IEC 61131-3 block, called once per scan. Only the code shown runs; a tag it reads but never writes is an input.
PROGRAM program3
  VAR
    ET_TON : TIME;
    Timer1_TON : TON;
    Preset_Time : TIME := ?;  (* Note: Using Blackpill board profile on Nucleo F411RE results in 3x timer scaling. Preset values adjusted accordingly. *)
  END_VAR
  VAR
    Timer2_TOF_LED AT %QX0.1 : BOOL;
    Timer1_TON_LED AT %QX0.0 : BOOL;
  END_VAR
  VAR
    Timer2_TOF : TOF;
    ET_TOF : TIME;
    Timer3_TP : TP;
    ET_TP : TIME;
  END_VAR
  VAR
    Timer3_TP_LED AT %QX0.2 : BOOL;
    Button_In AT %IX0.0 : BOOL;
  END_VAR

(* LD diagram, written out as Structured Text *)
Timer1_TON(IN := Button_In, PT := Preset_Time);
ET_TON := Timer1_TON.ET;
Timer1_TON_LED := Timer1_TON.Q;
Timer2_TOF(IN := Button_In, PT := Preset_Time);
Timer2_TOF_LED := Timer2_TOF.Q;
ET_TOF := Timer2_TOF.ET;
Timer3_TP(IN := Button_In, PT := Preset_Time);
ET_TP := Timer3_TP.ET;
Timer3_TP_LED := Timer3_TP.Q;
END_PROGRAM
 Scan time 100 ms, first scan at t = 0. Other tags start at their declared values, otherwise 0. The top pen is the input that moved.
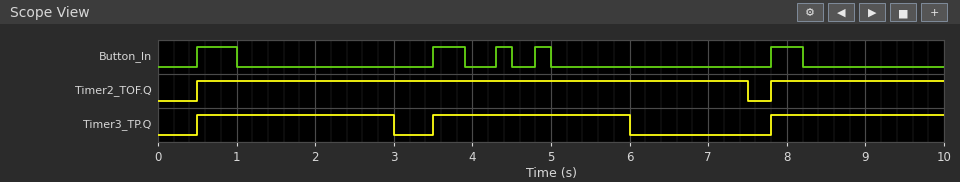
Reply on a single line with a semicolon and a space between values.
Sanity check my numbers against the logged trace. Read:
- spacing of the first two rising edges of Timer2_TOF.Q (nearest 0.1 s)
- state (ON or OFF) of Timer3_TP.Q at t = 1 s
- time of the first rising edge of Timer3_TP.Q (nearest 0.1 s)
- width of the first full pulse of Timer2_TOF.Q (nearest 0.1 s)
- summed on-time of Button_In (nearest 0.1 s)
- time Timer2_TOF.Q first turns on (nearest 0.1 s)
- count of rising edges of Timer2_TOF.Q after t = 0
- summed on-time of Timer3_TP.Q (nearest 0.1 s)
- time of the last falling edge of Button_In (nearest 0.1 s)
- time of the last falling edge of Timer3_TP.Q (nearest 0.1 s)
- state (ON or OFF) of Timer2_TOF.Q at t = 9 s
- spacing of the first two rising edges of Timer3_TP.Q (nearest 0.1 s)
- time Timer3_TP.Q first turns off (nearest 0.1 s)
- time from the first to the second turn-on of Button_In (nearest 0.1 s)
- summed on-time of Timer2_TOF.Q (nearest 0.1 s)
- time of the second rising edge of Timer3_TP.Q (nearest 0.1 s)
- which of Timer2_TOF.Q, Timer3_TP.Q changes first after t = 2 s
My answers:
7.3 s; ON; 0.5 s; 7.0 s; 1.7 s; 0.5 s; 2; 7.2 s; 8.2 s; 6.0 s; ON; 3.0 s; 3.0 s; 3.0 s; 9.2 s; 3.5 s; Timer3_TP.Q
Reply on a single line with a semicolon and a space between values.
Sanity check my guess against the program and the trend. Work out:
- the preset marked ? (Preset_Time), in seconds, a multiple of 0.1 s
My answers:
2.5 s
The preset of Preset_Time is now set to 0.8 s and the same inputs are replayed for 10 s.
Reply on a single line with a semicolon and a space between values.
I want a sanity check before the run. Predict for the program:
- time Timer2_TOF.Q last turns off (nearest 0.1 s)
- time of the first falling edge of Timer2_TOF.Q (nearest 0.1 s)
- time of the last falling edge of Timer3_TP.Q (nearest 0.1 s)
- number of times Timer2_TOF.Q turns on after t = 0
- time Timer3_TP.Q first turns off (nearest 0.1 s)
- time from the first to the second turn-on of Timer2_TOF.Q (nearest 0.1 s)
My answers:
9.0 s; 1.8 s; 8.6 s; 3; 1.3 s; 3.0 s
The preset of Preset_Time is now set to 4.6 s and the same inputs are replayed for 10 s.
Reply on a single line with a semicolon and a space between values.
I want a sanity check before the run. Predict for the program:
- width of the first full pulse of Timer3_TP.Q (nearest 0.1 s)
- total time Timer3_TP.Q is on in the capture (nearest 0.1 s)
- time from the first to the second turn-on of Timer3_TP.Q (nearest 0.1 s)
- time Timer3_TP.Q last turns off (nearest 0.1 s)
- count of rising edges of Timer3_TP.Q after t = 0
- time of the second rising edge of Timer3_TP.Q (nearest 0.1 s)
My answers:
4.6 s; 6.8 s; 7.3 s; 5.1 s; 2; 7.8 s
